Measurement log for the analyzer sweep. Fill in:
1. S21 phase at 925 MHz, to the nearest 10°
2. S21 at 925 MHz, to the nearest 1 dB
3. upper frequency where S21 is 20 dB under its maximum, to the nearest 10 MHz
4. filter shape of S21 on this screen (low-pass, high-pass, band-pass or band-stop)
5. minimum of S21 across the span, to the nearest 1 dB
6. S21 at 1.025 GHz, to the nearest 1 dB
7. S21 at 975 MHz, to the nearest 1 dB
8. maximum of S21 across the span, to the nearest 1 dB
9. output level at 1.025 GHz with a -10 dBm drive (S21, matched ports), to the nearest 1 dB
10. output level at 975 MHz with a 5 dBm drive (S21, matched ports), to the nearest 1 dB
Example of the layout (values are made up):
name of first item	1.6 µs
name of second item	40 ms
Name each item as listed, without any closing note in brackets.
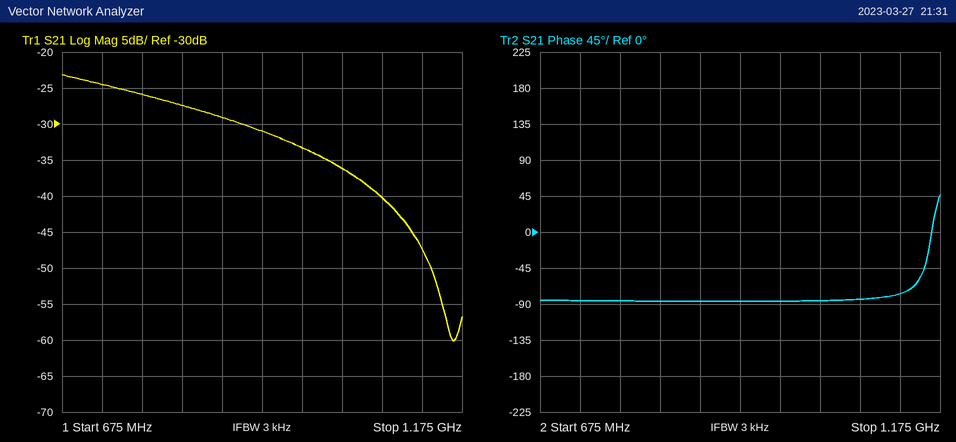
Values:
S21 phase at 925 MHz, to the nearest 10°	-90°
S21 at 925 MHz, to the nearest 1 dB	-31 dB
upper frequency where S21 is 20 dB under its maximum, to the nearest 10 MHz	1.10 GHz
filter shape of S21 on this screen	low-pass
minimum of S21 across the span, to the nearest 1 dB	-60 dB
S21 at 1.025 GHz, to the nearest 1 dB	-36 dB
S21 at 975 MHz, to the nearest 1 dB	-33 dB
maximum of S21 across the span, to the nearest 1 dB	-23 dB
output level at 1.025 GHz with a -10 dBm drive (S21, matched ports), to the nearest 1 dB	-46 dBm
output level at 975 MHz with a 5 dBm drive (S21, matched ports), to the nearest 1 dB	-28 dBm
